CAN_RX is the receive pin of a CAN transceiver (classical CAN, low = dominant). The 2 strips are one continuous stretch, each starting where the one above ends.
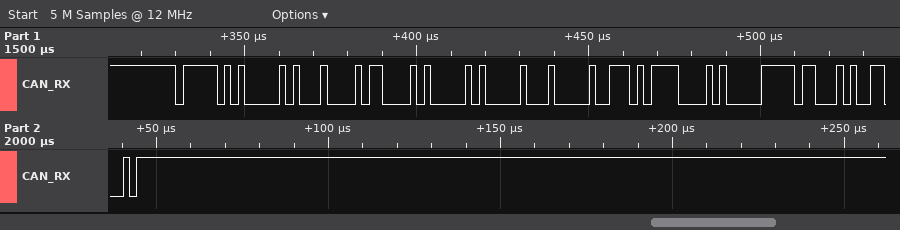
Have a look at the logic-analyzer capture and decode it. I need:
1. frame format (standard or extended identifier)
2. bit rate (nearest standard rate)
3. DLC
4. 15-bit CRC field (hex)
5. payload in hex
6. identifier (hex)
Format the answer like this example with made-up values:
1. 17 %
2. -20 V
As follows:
1. standard
2. 500 kbit/s
3. 8
4. 0x714C
5. 85 85 02 01 01 D7 85 07
6. 0x7E8
